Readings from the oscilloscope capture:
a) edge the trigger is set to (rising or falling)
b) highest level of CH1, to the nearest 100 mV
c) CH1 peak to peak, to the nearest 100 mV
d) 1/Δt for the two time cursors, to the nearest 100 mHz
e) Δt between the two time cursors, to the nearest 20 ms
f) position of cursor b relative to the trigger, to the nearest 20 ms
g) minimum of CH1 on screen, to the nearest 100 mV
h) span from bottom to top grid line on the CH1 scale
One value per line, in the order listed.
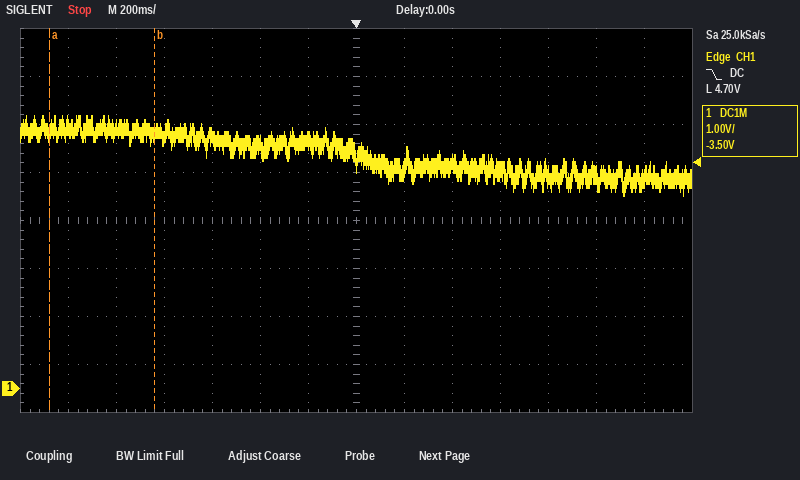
falling
5.7 V
1.7 V
2.3 Hz
440 ms
-840 ms
4.0 V
8 V
